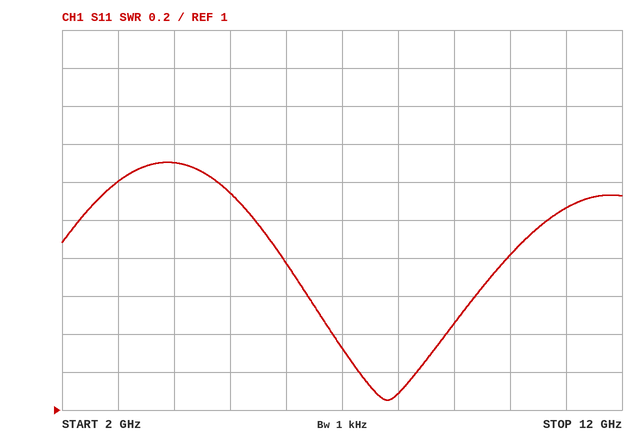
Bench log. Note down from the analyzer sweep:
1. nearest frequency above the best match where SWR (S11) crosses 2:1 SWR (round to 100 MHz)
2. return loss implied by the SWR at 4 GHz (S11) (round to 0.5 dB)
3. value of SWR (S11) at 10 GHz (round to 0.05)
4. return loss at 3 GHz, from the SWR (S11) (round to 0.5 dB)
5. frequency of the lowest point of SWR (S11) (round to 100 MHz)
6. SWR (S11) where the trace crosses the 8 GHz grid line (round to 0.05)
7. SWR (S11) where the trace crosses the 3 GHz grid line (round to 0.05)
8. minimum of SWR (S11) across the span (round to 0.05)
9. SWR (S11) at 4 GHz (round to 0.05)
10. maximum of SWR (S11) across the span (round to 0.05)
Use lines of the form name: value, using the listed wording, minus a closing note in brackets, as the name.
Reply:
nearest frequency above the best match where SWR (S11) crosses 2:1 SWR: 10.7 GHz
return loss implied by the SWR at 4 GHz (S11): 8.0 dB
value of SWR (S11) at 10 GHz: 1.80
return loss at 3 GHz, from the SWR (S11): 8.5 dB
frequency of the lowest point of SWR (S11): 7.8 GHz
SWR (S11) where the trace crosses the 8 GHz grid line: 1.10
SWR (S11) where the trace crosses the 3 GHz grid line: 2.20
minimum of SWR (S11) across the span: 1.05
SWR (S11) at 4 GHz: 2.30
maximum of SWR (S11) across the span: 2.30
